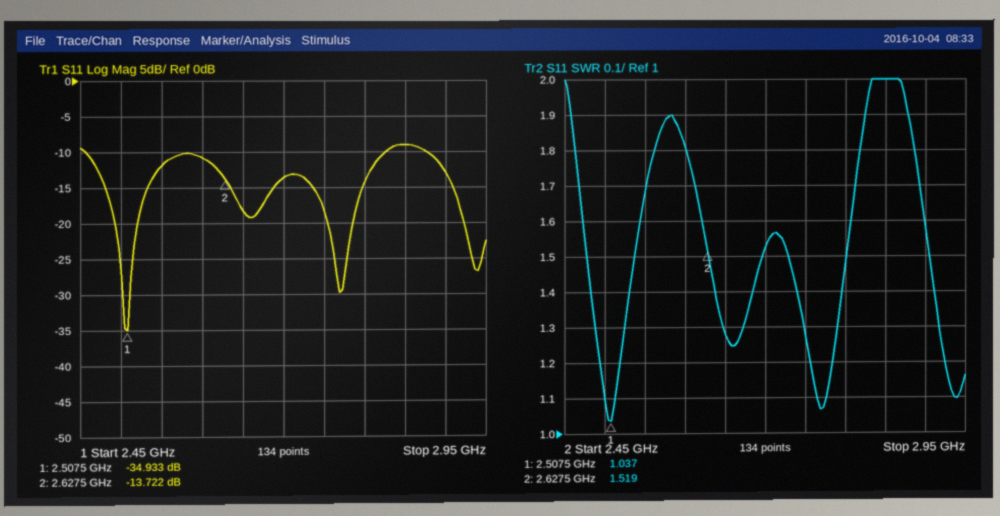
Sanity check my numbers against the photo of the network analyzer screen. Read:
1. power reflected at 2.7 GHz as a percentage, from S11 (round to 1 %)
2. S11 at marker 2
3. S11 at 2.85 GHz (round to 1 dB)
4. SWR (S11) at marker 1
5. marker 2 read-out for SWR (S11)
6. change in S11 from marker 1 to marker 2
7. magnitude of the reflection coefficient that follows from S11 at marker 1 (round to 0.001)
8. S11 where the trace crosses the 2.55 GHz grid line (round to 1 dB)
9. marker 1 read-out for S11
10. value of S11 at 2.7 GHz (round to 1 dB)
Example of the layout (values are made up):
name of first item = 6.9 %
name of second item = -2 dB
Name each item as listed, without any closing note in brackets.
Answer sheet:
power reflected at 2.7 GHz as a percentage, from S11 = 4 %
S11 at marker 2 = -13.722 dB
S11 at 2.85 GHz = -9 dB
SWR (S11) at marker 1 = 1.037
marker 2 read-out for SWR = 1.519
change in S11 from marker 1 to marker 2 = 21.211 dB
magnitude of the reflection coefficient that follows from S11 at marker 1 = 0.018
S11 where the trace crosses the 2.55 GHz grid line = -12 dB
marker 1 read-out for S11 = -34.933 dB
value of S11 at 2.7 GHz = -14 dB
